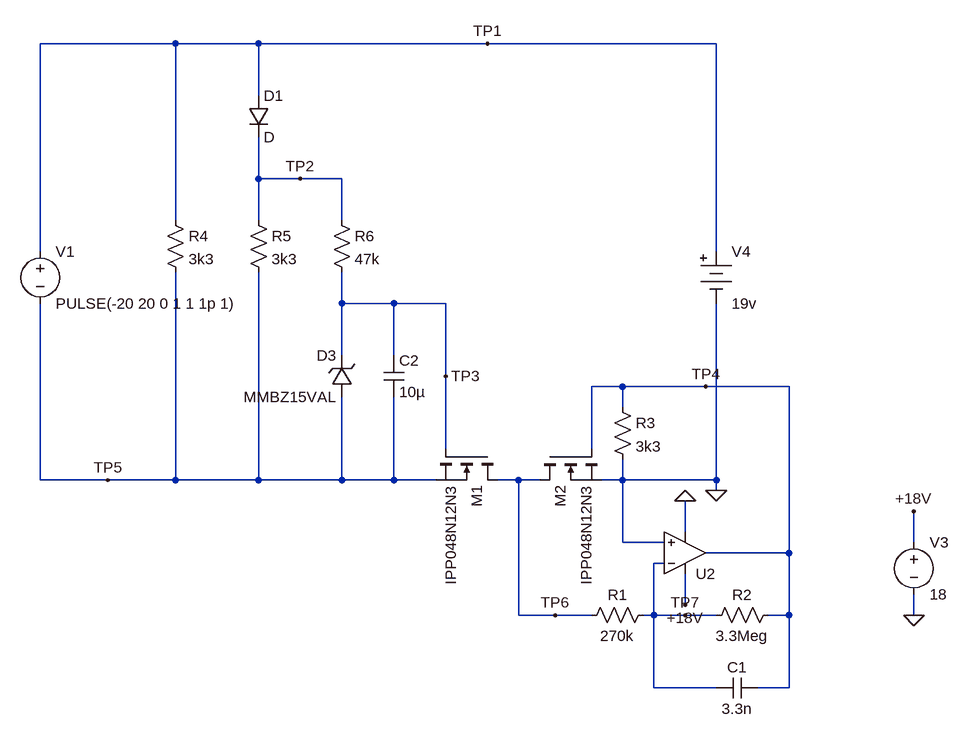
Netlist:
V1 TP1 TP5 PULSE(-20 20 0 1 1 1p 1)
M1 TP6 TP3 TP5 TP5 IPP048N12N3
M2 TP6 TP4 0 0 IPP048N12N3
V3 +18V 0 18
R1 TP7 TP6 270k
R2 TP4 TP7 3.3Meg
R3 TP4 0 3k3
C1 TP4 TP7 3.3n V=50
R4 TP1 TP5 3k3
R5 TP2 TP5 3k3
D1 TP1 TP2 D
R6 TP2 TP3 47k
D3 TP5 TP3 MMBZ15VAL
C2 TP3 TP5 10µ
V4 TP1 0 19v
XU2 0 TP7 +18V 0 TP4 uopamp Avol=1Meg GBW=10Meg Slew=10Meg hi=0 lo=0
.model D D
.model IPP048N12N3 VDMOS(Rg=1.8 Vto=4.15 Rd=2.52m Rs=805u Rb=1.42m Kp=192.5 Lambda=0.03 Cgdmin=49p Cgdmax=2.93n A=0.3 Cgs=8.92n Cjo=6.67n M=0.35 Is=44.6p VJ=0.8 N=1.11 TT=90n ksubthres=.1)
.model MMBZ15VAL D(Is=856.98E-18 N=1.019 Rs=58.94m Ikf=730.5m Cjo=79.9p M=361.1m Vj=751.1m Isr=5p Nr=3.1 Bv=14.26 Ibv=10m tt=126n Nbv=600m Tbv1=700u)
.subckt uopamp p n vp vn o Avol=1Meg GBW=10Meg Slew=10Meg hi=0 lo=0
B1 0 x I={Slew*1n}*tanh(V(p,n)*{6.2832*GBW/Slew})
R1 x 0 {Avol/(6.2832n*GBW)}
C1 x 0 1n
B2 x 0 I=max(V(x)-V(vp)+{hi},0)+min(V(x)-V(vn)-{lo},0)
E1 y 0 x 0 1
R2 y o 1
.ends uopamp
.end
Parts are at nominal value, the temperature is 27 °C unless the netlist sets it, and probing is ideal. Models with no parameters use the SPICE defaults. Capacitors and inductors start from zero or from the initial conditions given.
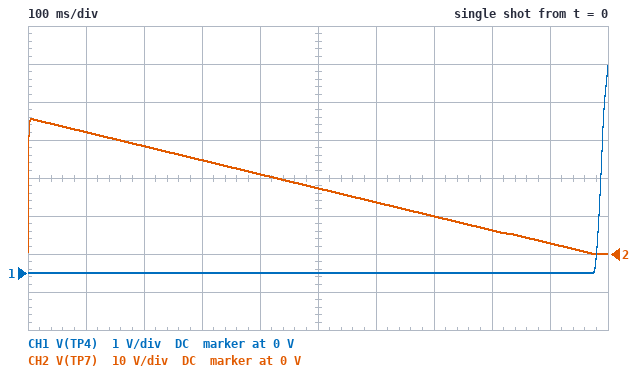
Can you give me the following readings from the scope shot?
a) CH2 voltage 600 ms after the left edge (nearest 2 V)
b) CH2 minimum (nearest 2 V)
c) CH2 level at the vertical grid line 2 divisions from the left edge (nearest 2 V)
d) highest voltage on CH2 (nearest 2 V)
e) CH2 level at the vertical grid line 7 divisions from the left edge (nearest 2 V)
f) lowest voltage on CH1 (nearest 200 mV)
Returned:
14 V
0 V
28 V
36 V
10 V
0 V
